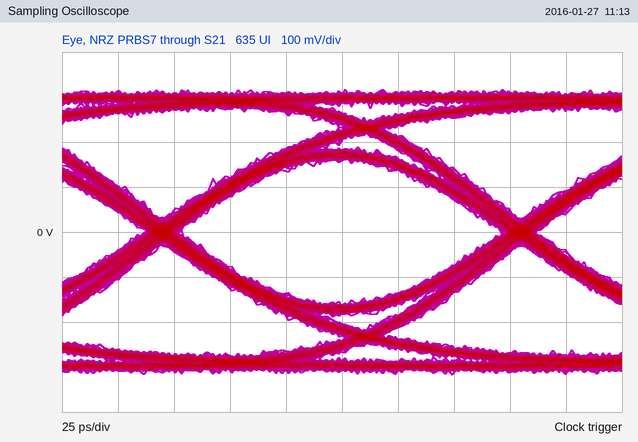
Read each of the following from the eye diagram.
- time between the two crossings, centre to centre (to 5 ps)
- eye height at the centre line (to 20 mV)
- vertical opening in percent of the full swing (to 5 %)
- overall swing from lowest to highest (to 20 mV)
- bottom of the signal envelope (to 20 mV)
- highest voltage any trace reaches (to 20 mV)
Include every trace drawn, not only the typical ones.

160 ps
320 mV
50 %
640 mV
-320 mV
320 mV
